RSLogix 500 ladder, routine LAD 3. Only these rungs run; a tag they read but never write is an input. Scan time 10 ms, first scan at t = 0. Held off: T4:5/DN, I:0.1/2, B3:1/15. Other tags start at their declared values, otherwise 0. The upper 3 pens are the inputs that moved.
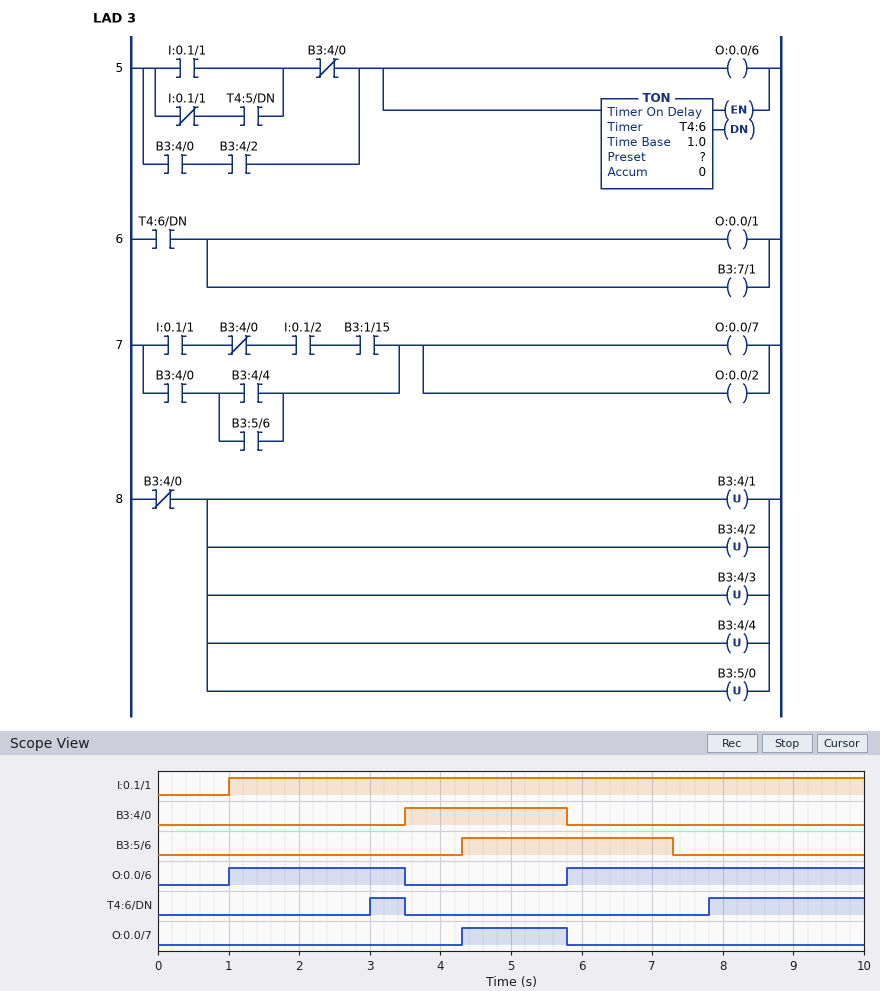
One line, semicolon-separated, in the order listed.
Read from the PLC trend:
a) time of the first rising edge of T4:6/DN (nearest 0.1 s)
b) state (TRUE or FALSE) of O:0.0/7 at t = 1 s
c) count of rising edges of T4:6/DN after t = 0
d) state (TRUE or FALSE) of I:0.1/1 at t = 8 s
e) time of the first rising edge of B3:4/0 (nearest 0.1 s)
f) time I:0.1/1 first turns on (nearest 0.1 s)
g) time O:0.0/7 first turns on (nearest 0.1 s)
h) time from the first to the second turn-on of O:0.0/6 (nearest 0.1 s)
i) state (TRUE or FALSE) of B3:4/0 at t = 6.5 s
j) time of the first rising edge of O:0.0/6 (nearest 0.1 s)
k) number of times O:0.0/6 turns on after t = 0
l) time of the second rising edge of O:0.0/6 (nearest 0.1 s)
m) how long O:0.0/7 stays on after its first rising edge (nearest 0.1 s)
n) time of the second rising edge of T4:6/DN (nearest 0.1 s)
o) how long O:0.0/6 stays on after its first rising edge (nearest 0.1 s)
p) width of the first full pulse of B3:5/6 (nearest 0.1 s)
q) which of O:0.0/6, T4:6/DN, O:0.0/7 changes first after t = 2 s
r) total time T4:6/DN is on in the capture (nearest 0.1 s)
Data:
3.0 s; FALSE; 2; TRUE; 3.5 s; 1.0 s; 4.3 s; 4.8 s; FALSE; 1.0 s; 2; 5.8 s; 1.5 s; 7.8 s; 2.5 s; 3.0 s; T4:6/DN; 2.7 s
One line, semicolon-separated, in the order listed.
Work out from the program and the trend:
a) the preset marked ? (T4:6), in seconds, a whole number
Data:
2 s
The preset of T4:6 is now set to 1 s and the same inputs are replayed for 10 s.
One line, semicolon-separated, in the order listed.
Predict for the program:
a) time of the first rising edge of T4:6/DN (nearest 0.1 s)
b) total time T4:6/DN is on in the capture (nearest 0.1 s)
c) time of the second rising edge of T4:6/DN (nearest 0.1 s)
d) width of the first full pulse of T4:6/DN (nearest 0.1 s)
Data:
2.0 s; 4.7 s; 6.8 s; 1.5 s
